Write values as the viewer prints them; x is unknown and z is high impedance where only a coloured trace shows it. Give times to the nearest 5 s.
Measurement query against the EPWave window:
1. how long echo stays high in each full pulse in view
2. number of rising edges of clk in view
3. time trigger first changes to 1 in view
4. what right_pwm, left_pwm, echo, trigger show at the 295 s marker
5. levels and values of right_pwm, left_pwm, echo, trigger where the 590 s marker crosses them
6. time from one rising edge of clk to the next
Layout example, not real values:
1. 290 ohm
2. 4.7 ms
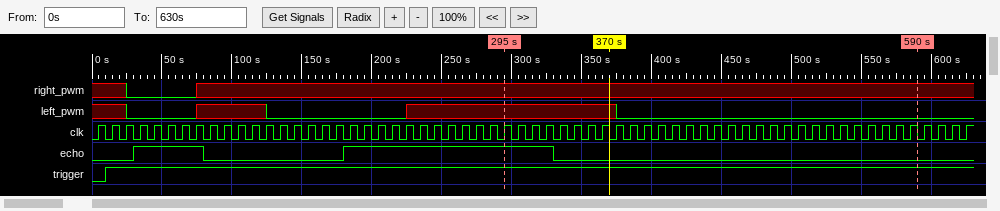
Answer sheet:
1. 50 s, 150 s
2. 63
3. 10 s
4. right_pwm=x, left_pwm=x, echo=1, trigger=1
5. right_pwm=x, left_pwm=0, echo=0, trigger=1
6. 10 s
